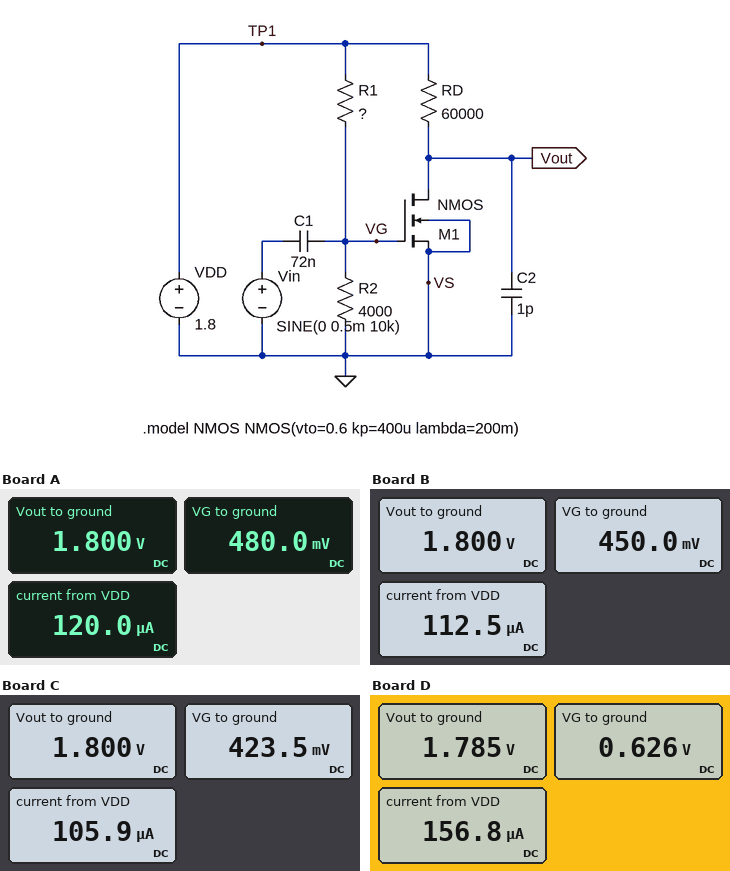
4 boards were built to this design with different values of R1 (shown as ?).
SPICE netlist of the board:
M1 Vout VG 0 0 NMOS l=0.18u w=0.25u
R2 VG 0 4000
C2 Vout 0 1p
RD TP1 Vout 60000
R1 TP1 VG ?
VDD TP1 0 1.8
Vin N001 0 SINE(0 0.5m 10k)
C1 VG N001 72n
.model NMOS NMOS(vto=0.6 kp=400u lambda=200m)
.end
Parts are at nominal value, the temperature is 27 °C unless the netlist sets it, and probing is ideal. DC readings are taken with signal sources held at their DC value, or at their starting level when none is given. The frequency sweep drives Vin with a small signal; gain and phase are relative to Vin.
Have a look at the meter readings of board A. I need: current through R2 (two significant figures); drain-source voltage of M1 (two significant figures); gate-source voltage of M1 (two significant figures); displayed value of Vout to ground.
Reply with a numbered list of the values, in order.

1. 120 µA
2. 1.8 V
3. 480 mV
4. 1.800 V
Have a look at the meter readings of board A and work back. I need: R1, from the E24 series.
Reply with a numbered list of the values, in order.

1. 11 kΩ
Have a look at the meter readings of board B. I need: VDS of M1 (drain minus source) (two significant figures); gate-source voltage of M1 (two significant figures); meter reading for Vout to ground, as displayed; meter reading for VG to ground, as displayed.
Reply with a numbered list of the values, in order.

1. 1.8 V
2. 450 mV
3. 1.800 V
4. 450.0 mV
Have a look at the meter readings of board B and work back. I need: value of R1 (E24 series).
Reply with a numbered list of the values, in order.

1. 12 kΩ
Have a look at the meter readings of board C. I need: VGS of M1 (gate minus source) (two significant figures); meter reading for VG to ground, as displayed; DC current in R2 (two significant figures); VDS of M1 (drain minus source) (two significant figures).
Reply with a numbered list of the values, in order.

1. 420 mV
2. 423.5 mV
3. 110 µA
4. 1.8 V
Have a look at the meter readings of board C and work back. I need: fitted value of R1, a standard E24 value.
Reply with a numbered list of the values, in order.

1. 13 kΩ
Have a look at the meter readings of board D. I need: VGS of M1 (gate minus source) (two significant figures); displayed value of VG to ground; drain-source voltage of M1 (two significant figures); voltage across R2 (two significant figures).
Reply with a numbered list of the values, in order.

1. 630 mV
2. 0.626 V
3. 1.8 V
4. 630 mV
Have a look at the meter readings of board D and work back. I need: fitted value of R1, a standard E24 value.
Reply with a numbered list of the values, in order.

1. 7.5 kΩ
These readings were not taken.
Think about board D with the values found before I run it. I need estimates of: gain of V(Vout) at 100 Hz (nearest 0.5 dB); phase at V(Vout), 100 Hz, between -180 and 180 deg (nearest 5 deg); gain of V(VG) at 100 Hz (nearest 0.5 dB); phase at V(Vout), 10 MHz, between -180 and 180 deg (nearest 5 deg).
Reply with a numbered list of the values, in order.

1. -17.0 dB
2. -95 deg
3. -18.5 dB
4. 105 deg
